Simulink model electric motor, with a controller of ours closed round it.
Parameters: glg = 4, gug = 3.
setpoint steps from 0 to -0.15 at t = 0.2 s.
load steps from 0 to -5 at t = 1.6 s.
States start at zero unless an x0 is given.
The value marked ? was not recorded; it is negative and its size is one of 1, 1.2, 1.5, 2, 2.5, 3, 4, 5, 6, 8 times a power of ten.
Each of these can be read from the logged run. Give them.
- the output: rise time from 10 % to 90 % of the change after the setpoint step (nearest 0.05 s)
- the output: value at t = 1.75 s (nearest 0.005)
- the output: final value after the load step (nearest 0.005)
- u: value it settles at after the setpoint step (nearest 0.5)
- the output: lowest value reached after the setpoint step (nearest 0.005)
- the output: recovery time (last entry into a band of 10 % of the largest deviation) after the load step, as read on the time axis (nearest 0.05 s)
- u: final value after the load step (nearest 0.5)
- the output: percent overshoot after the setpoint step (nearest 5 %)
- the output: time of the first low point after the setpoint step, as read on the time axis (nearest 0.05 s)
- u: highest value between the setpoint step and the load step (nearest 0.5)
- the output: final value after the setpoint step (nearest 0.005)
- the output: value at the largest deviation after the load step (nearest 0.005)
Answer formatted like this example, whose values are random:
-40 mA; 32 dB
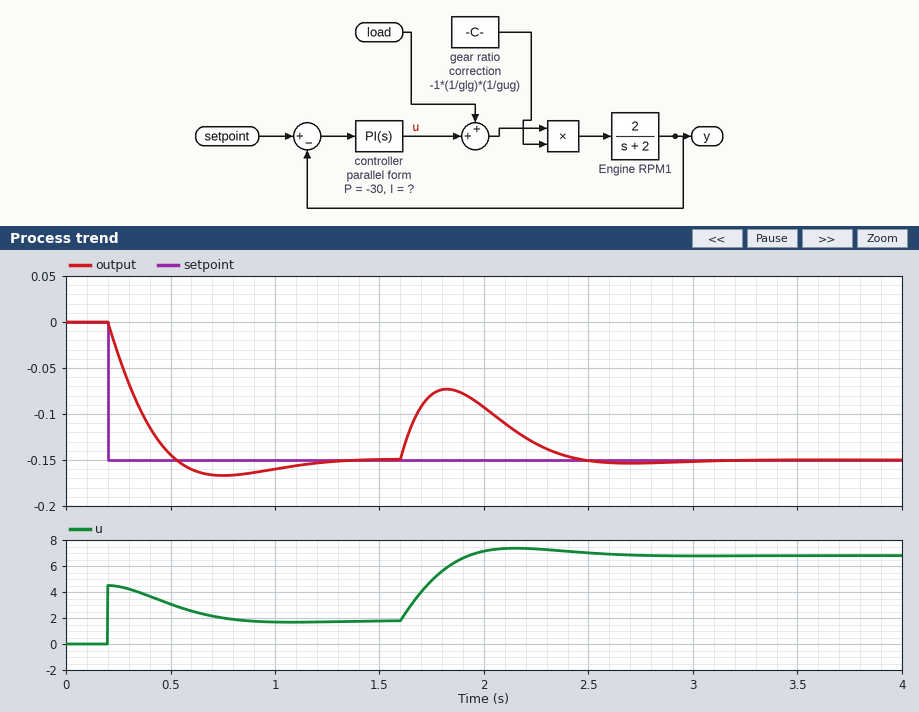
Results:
0.25 s; -0.080; -0.150; 2.0; -0.165; 2.35 s; 7.0; 10 %; 0.75 s; 4.5; -0.150; -0.075
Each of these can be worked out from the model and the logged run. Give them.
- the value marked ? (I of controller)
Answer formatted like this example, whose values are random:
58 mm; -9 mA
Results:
-150
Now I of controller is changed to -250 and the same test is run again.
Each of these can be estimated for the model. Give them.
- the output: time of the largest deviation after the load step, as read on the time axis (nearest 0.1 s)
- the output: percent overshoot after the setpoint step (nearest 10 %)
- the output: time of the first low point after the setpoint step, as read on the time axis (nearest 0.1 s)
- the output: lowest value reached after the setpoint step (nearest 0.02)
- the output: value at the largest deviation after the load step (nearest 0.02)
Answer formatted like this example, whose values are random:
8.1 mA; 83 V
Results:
1.8 s; 20 %; 0.6 s; -0.18; -0.08
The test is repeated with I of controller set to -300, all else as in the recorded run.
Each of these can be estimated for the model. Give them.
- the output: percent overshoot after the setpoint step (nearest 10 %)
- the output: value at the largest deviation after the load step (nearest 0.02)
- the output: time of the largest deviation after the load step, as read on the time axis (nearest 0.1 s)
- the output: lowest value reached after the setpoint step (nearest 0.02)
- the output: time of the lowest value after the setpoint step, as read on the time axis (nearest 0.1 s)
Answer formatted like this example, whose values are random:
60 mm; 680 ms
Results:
20 %; -0.08; 1.8 s; -0.18; 0.6 s
